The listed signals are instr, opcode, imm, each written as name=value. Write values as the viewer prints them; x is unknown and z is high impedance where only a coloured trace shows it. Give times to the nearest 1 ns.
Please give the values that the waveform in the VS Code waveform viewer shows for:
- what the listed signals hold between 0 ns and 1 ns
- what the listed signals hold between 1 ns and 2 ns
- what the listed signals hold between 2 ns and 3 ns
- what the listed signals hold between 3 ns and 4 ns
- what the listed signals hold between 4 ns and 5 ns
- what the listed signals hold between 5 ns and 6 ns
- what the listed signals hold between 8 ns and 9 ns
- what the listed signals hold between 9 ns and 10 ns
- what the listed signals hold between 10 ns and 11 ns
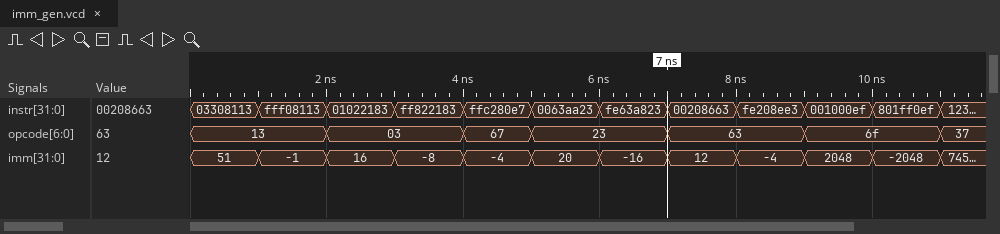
instr=03308113, opcode=13, imm=51
instr=fff08113, opcode=13, imm=-1
instr=01022183, opcode=03, imm=16
instr=ff822183, opcode=03, imm=-8
instr=ffc280e7, opcode=67, imm=-4
instr=0063aa23, opcode=23, imm=20
instr=fe208ee3, opcode=63, imm=-4
instr=001000ef, opcode=6f, imm=2048
instr=801ff0ef, opcode=6f, imm=-2048
